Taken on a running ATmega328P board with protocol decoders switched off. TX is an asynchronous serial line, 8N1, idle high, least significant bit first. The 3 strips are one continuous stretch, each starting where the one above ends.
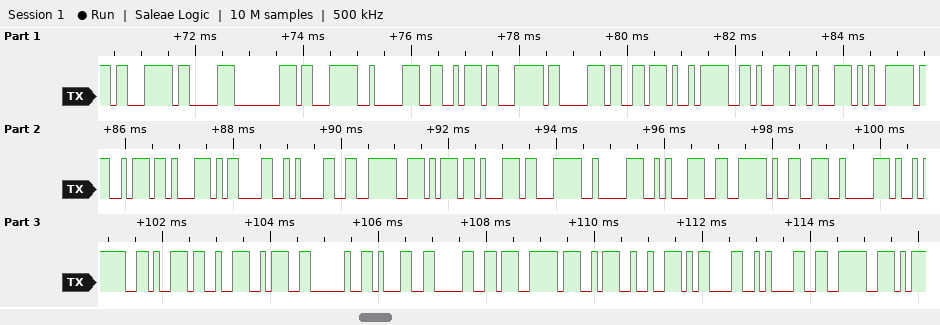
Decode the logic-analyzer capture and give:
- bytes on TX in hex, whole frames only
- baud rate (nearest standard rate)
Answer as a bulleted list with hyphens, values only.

- 0xE3 0x83 0x80 0xE3 0x82 0xA6 0xE3 0x83 0xB3 0xE9 0x96 0x8B 0xE5 0xA7 0x8B 0x0D 0x0A 0xE6 0xAE 0x8B 0xE3 0x82 0x8A 0xE6 0x99 0x82 0xE9 0x96 0x93 0x3A 0x20 0x31 0x30 0xE7 0xA7 0x92 0x0D 0x0A 0xE6 0xAE
- 9600 baud
